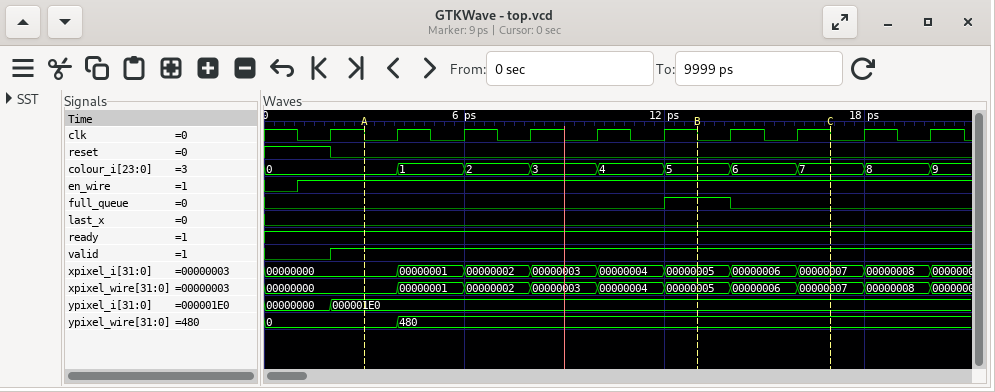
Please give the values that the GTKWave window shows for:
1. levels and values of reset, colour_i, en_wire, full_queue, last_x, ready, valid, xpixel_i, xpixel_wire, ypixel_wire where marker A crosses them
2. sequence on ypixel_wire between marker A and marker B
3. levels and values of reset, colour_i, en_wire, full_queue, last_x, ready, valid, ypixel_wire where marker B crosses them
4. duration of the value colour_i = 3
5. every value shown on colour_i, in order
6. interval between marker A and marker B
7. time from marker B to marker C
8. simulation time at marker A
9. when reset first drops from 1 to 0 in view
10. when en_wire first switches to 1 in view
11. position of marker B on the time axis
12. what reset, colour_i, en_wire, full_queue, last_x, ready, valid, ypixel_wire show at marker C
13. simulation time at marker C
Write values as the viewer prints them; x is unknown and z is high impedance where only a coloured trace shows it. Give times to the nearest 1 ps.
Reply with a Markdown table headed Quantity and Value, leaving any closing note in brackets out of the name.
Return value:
| Quantity | Value |
|---|---|
| levels and values of reset, colour_i, en_wire, full_queue, last_x, ready, valid, xpixel_i, xpixel_wire, ypixel_wire where marker A crosses them | reset=0, colour_i=0, en_wire=1, full_queue=0, last_x=0, ready=1, valid=1, xpixel_i=00000000, xpixel_wire=00000000, ypixel_wire=0 |
| sequence on ypixel_wire between marker A and marker B | 0, 480 |
| levels and values of reset, colour_i, en_wire, full_queue, last_x, ready, valid, ypixel_wire where marker B crosses them | reset=0, colour_i=5, en_wire=1, full_queue=1, last_x=0, ready=1, valid=1, ypixel_wire=480 |
| duration of the value colour_i = 3 | 2 ps |
| every value shown on colour_i, in order | 0, 1, 2, 3, 4, 5, 6, 7, 8, 9 |
| interval between marker A and marker B | 10 ps |
| time from marker B to marker C | 4 ps |
| simulation time at marker A | 3 ps |
| when reset first drops from 1 to 0 in view | 2 ps |
| when en_wire first switches to 1 in view | 1 ps |
| position of marker B on the time axis | 13 ps |
| what reset, colour_i, en_wire, full_queue, last_x, ready, valid, ypixel_wire show at marker C | reset=0, colour_i=7, en_wire=1, full_queue=0, last_x=0, ready=1, valid=1, ypixel_wire=480 |
| simulation time at marker C | 17 ps |
